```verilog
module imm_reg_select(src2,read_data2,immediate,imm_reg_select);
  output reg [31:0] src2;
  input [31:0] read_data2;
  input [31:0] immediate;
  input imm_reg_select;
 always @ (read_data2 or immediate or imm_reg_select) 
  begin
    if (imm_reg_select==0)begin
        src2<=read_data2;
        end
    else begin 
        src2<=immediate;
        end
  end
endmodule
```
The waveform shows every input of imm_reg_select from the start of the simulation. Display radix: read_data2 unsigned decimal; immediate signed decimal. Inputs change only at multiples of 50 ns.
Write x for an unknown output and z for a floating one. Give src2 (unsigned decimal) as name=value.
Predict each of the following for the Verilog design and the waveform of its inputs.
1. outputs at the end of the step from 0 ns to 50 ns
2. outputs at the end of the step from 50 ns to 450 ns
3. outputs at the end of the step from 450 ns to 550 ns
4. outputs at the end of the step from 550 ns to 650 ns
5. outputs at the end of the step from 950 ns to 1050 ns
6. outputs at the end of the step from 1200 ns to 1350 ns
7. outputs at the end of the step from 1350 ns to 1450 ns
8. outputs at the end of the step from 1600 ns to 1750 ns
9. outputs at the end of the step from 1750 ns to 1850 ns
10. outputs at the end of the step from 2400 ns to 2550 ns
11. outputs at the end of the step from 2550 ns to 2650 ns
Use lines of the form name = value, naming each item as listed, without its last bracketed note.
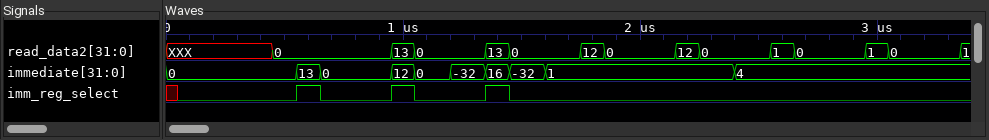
outputs at the end of the step from 0 ns to 50 ns = src2=0
outputs at the end of the step from 50 ns to 450 ns = src2=x
outputs at the end of the step from 450 ns to 550 ns = src2=0
outputs at the end of the step from 550 ns to 650 ns = src2=13
outputs at the end of the step from 950 ns to 1050 ns = src2=12
outputs at the end of the step from 1200 ns to 1350 ns = src2=0
outputs at the end of the step from 1350 ns to 1450 ns = src2=16
outputs at the end of the step from 1600 ns to 1750 ns = src2=0
outputs at the end of the step from 1750 ns to 1850 ns = src2=12
outputs at the end of the step from 2400 ns to 2550 ns = src2=0
outputs at the end of the step from 2550 ns to 2650 ns = src2=1
